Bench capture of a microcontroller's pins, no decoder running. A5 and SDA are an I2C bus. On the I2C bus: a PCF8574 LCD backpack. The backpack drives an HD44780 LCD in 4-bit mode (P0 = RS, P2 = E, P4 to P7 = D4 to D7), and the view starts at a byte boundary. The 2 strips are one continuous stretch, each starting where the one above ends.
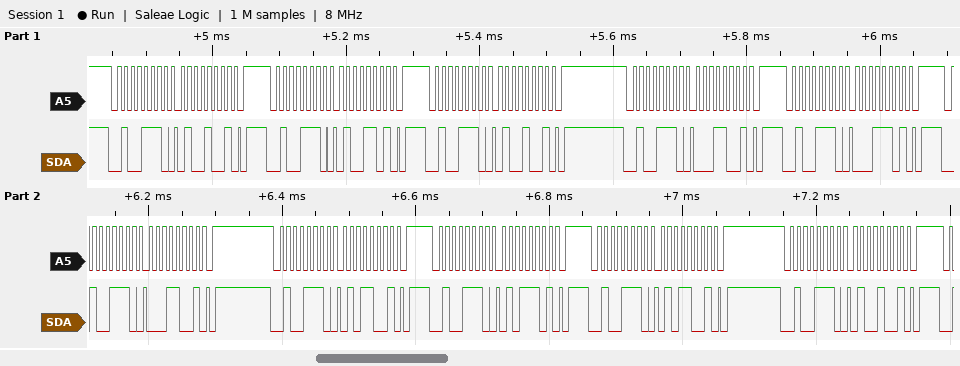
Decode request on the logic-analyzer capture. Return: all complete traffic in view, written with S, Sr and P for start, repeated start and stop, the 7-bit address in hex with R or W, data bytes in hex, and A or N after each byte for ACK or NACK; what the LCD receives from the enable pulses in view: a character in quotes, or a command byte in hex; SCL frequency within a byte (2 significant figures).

S 27W A 49 A P S 27W A 4D A P S 27W A 49 A P S 27W A 19 A P S 27W A 1D A P S 27W A 19 A P S 27W A 59 A P S 27W A 5D A P S 27W A 59 A P S 27W A 49 A P
'A'
100 kHz
